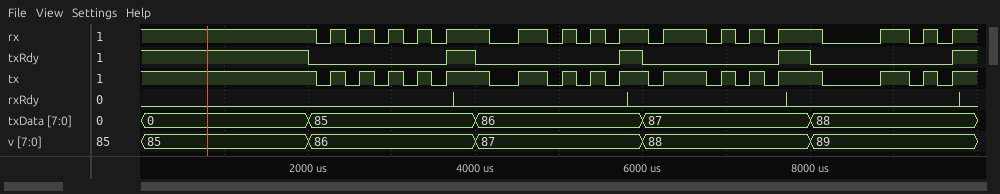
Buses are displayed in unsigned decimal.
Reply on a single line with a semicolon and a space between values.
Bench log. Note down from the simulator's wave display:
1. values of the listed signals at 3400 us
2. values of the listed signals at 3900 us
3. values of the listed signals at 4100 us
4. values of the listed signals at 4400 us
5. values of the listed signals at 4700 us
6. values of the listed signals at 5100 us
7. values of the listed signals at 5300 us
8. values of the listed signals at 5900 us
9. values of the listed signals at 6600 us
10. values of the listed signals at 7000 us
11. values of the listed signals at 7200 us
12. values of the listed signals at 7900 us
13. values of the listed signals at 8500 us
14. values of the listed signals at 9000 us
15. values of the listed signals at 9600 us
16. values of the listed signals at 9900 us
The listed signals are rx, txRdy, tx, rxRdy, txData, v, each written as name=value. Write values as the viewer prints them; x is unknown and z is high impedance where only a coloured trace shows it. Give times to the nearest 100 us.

rx=1, txRdy=0, tx=1, rxRdy=0, txData=85, v=86; rx=1, txRdy=1, tx=1, rxRdy=0, txData=85, v=86; rx=1, txRdy=0, tx=1, rxRdy=0, txData=86, v=87; rx=0, txRdy=0, tx=0, rxRdy=0, txData=86, v=87; rx=1, txRdy=0, tx=1, rxRdy=0, txData=86, v=87; rx=1, txRdy=0, tx=1, rxRdy=0, txData=86, v=87; rx=0, txRdy=0, tx=0, rxRdy=0, txData=86, v=87; rx=1, txRdy=1, tx=1, rxRdy=0, txData=86, v=87; rx=1, txRdy=0, tx=1, rxRdy=0, txData=87, v=88; rx=1, txRdy=0, tx=1, rxRdy=0, txData=87, v=88; rx=0, txRdy=0, tx=0, rxRdy=0, txData=87, v=88; rx=1, txRdy=1, tx=1, rxRdy=0, txData=87, v=88; rx=0, txRdy=0, tx=0, rxRdy=0, txData=88, v=89; rx=1, txRdy=0, tx=1, rxRdy=0, txData=88, v=89; rx=0, txRdy=0, tx=0, rxRdy=0, txData=88, v=89; rx=1, txRdy=1, tx=1, rxRdy=0, txData=88, v=89
